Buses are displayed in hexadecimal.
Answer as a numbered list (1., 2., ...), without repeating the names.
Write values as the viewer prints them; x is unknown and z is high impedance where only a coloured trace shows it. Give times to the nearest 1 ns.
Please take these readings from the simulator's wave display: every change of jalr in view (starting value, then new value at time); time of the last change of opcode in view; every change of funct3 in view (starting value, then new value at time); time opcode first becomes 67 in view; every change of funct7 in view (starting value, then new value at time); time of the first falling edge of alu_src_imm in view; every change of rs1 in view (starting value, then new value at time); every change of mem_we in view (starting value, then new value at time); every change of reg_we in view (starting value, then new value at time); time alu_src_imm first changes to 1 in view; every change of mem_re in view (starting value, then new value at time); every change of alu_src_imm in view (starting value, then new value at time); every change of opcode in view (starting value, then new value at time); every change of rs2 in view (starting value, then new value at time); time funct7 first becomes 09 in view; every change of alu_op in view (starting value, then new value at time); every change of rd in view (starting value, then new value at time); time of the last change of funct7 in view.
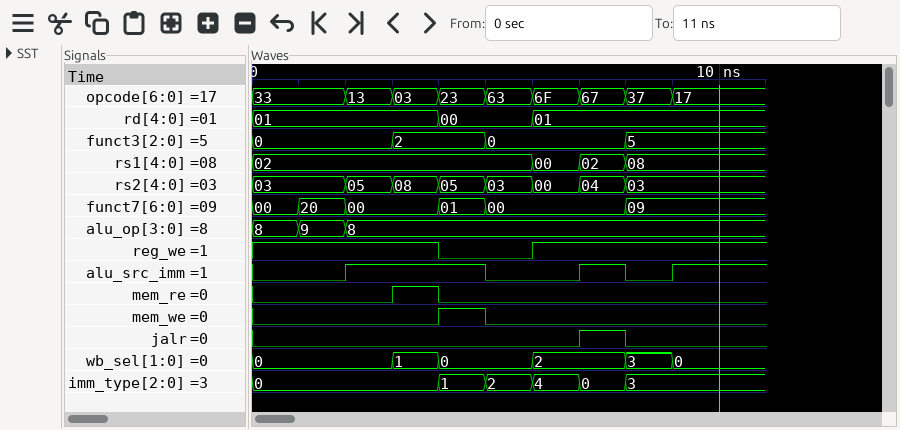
1. 0, 1 at 7 ns, 0 at 8 ns
2. 9 ns
3. 0, 2 at 3 ns, 0 at 5 ns, 5 at 8 ns
4. 7 ns
5. 00, 20 at 1 ns, 00 at 2 ns, 01 at 4 ns, 00 at 5 ns, 09 at 8 ns
6. 5 ns
7. 02, 00 at 6 ns, 02 at 7 ns, 08 at 8 ns
8. 0, 1 at 4 ns, 0 at 5 ns
9. 1, 0 at 4 ns, 1 at 6 ns
10. 2 ns
11. 0, 1 at 3 ns, 0 at 4 ns
12. 0, 1 at 2 ns, 0 at 5 ns, 1 at 7 ns, 0 at 8 ns, 1 at 9 ns
13. 33, 13 at 2 ns, 03 at 3 ns, 23 at 4 ns, 63 at 5 ns, 6F at 6 ns, 67 at 7 ns, 37 at 8 ns, 17 at 9 ns
14. 03, 05 at 2 ns, 08 at 3 ns, 05 at 4 ns, 03 at 5 ns, 00 at 6 ns, 04 at 7 ns, 03 at 8 ns
15. 8 ns
16. 8, 9 at 1 ns, 8 at 2 ns
17. 01, 00 at 4 ns, 01 at 6 ns
18. 8 ns
